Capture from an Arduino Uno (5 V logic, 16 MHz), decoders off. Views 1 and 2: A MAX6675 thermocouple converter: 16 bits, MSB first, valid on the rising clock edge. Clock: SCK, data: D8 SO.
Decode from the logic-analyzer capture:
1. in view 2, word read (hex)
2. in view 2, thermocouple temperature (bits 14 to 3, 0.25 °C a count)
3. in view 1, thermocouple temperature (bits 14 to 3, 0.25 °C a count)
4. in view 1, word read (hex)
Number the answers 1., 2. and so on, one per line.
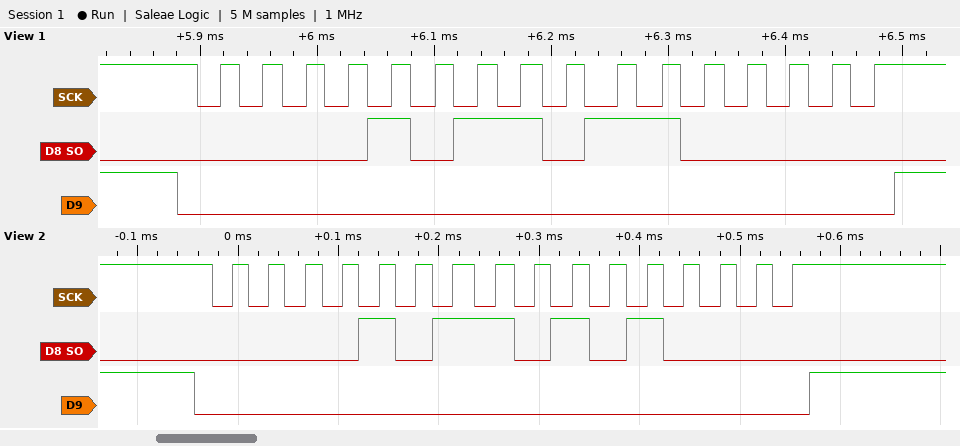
1. 0x0B50
2. 90.50 °C
3. 91.00 °C
4. 0x0B60
